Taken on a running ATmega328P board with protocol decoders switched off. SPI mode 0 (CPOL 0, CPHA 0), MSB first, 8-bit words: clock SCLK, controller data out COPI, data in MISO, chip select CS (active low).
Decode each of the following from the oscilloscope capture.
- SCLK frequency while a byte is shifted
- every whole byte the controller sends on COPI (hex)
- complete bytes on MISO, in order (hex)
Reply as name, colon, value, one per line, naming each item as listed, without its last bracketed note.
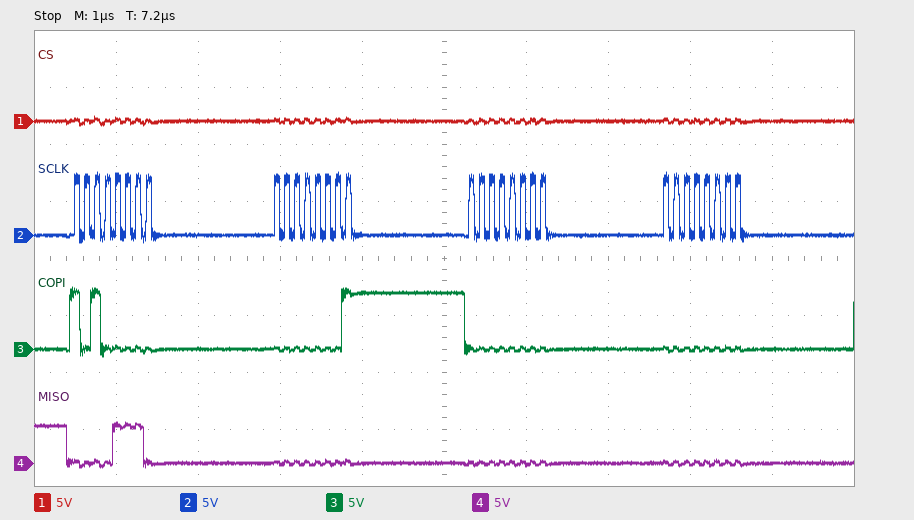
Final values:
SCLK frequency while a byte is shifted: 8 MHz
every whole byte the controller sends on COPI: A0 01 00 00
complete bytes on MISO, in order: 0E 00 00 00
